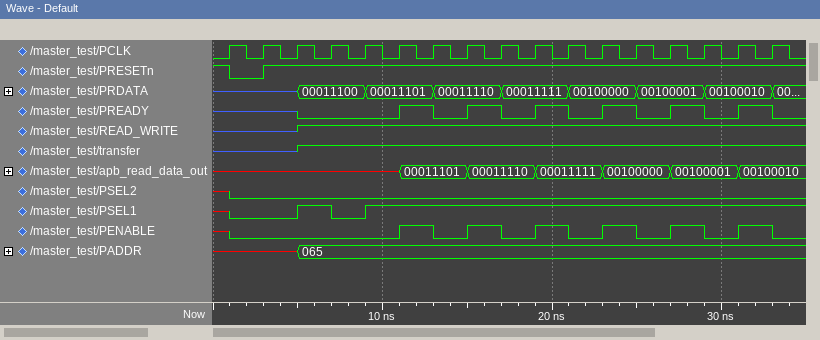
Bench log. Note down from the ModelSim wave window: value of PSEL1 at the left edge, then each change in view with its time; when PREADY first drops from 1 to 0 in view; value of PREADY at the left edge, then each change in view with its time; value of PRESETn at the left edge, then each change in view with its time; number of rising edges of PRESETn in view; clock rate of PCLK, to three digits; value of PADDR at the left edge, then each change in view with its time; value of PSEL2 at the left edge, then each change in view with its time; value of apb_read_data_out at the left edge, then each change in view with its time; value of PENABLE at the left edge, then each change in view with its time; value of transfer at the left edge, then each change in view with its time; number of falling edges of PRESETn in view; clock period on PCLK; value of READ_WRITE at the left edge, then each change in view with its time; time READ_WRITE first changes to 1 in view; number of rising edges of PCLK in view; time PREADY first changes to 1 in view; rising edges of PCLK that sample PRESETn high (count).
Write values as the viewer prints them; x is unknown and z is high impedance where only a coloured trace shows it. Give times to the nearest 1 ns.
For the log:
x, 0 at 1 ns, 1 at 5 ns, 0 at 7 ns, 1 at 9 ns
13 ns
z, 0 at 5 ns, 1 at 11 ns, 0 at 13 ns, 1 at 15 ns, 0 at 17 ns, 1 at 19 ns, 0 at 21 ns, 1 at 23 ns, 0 at 25 ns, 1 at 27 ns, 0 at 29 ns, 1 at 31 ns, 0 at 33 ns
1, 0 at 1 ns, 1 at 3 ns
1
500 MHz
x, 065 at 5 ns
x, 0 at 1 ns
x, 00011101 at 11 ns, 00011110 at 15 ns, 00011111 at 19 ns, 00100000 at 23 ns, 00100001 at 27 ns, 00100010 at 31 ns
x, 0 at 1 ns, 1 at 11 ns, 0 at 13 ns, 1 at 15 ns, 0 at 17 ns, 1 at 19 ns, 0 at 21 ns, 1 at 23 ns, 0 at 25 ns, 1 at 27 ns, 0 at 29 ns, 1 at 31 ns, 0 at 33 ns
z, 1 at 5 ns
1
2 ns
z, 1 at 5 ns
5 ns
17
11 ns
16
